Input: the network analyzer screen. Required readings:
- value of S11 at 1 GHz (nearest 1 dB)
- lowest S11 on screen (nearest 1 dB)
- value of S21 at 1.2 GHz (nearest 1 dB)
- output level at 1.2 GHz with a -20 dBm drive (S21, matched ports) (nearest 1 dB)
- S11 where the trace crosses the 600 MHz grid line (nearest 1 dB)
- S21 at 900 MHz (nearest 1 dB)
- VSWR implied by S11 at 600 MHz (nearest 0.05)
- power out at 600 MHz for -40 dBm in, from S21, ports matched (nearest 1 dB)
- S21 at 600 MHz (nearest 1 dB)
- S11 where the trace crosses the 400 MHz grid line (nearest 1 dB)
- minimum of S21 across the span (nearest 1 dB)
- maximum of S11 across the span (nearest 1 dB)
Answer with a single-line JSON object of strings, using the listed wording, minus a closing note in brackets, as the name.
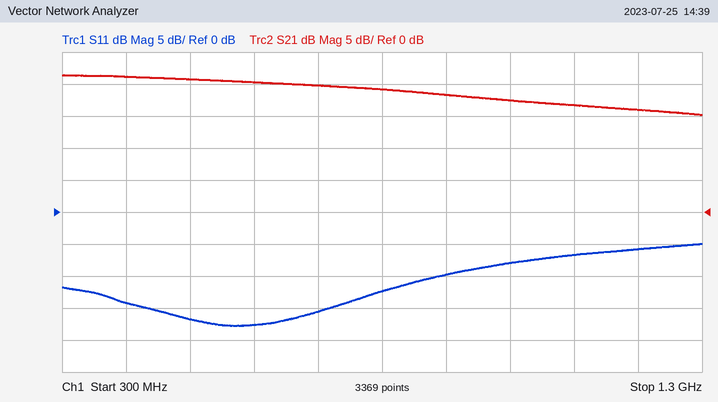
{"value of S11 at 1 GHz": "-8 dB", "lowest S11 on screen": "-18 dB", "value of S21 at 1.2 GHz": "16 dB", "output level at 1.2 GHz with a -20 dBm drive (S21, matched ports)": "-4 dBm", "S11 where the trace crosses the 600 MHz grid line": "-18 dB", "S21 at 900 MHz": "18 dB", "VSWR implied by S11 at 600 MHz": "1.30", "power out at 600 MHz for -40 dBm in, from S21, ports matched": "-20 dBm", "S21 at 600 MHz": "20 dB", "S11 where the trace crosses the 400 MHz grid line": "-14 dB", "minimum of S21 across the span": "15 dB", "maximum of S11 across the span": "-5 dB"}
